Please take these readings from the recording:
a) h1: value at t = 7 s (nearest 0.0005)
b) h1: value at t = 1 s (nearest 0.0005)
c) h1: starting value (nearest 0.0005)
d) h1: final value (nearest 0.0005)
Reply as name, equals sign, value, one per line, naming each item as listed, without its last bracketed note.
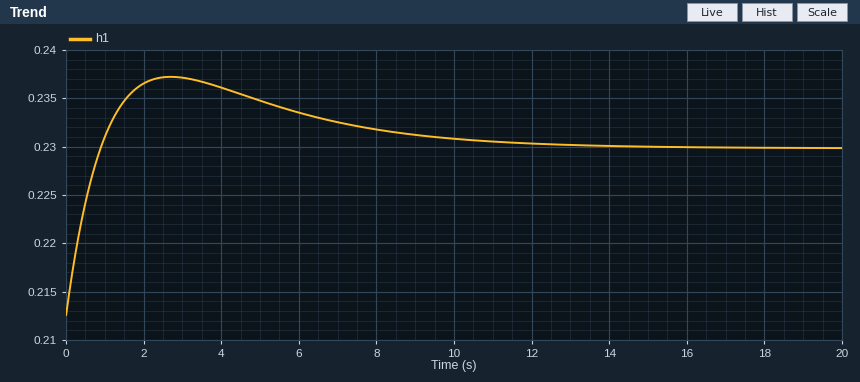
h1: value at t = 7 s = 0.2325
h1: value at t = 1 s = 0.2310
h1: starting value = 0.2125
h1: final value = 0.2300
